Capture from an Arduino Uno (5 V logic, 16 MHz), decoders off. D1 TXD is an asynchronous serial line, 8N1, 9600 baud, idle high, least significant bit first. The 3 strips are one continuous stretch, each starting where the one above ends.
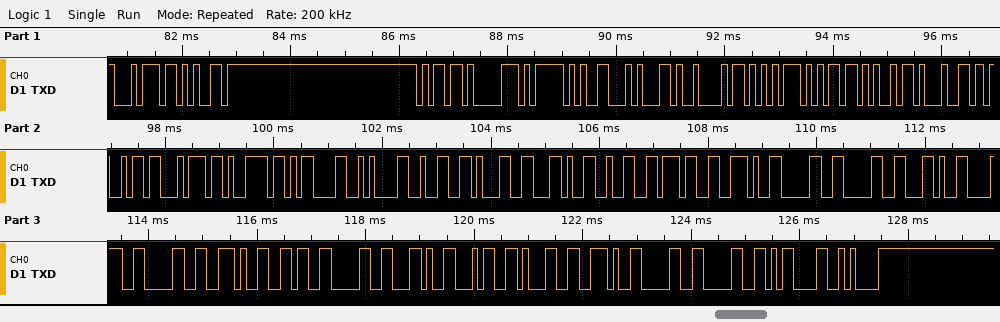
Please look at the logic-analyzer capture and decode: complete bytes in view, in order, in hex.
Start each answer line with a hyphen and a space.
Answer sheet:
- 0x74 0x65 0x6D 0x70 0x5F 0x46 0x2C 0x68 0x75 0x6D 0x69 0x64 0x69 0x74 0x79 0x0D 0x0A 0x32 0x31 0x2C 0x32 0x37 0x2E 0x30 0x30 0x2C 0x38 0x30 0x2E 0x36 0x30 0x2C 0x34 0x31 0x2E 0x30 0x30 0x0D 0x0A
